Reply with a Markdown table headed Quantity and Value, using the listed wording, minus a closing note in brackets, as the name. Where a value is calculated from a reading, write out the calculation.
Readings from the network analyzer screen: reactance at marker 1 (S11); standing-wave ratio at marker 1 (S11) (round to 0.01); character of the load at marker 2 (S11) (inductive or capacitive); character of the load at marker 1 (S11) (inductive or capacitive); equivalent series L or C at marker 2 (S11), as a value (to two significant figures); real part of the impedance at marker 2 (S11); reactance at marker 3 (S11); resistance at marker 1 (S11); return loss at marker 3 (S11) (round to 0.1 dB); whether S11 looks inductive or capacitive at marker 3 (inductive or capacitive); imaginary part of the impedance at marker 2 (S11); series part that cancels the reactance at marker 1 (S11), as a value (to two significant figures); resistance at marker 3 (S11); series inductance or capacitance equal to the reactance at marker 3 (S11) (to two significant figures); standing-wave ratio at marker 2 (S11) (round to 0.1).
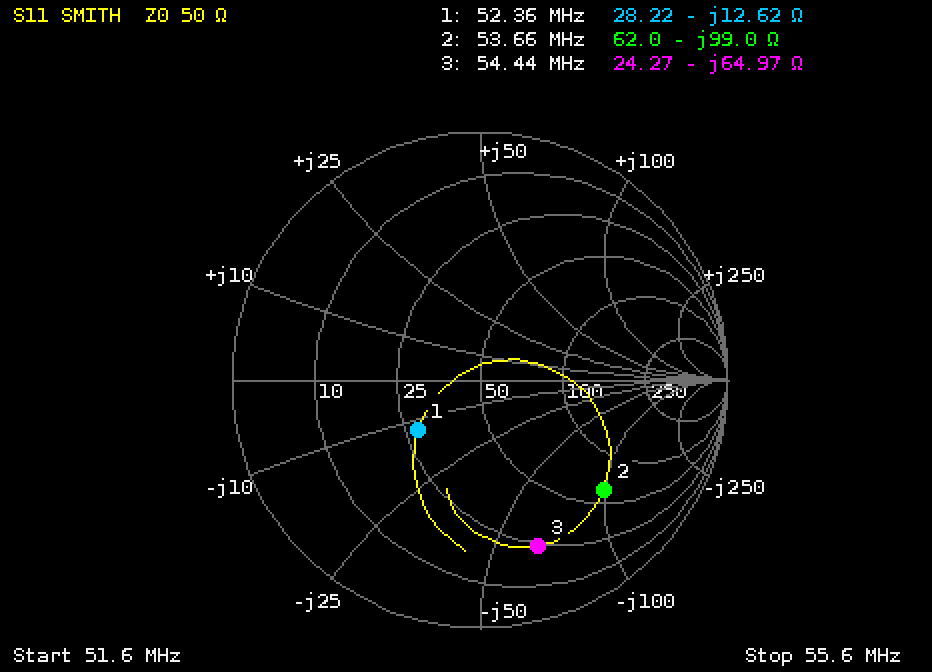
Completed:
| Quantity | Value |
|---|---|
| reactance at marker 1 | -12.62 Ω |
| standing-wave ratio at marker 1 (S11) | 1.93 |
| character of the load at marker 2 (S11) | capacitive |
| character of the load at marker 1 (S11) | capacitive |
| equivalent series L or C at marker 2 (S11), as a value | C = 1/(2π × 53.66 MHz × 99 Ω) ≈ 30 pF |
| real part of the impedance at marker 2 | 62.0 Ω |
| reactance at marker 3 | -64.97 Ω |
| resistance at marker 1 | 28.22 Ω |
| return loss at marker 3 (S11) | 3.0 dB |
| whether S11 looks inductive or capacitive at marker 3 | capacitive |
| imaginary part of the impedance at marker 2 | -99.0 Ω |
| series part that cancels the reactance at marker 1 (S11), as a value | L = 12.62 Ω/(2π × 52.36 MHz) ≈ 38 nH |
| resistance at marker 3 | 24.27 Ω |
| series inductance or capacitance equal to the reactance at marker 3 (S11) | C = 1/(2π × 54.44 MHz × 64.97 Ω) ≈ 45 pF |
| standing-wave ratio at marker 2 (S11) | 5.0 |
